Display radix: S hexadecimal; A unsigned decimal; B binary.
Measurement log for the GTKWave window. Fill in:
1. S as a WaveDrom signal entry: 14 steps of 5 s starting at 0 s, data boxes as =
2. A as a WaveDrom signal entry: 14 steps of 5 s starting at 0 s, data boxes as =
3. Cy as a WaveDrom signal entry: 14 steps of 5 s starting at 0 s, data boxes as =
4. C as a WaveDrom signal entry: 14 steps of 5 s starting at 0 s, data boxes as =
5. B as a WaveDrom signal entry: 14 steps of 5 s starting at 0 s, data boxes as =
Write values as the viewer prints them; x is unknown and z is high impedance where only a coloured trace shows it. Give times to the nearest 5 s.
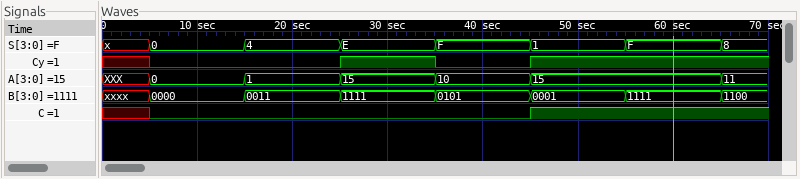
{name: 'S', wave: 'x=.=.=.=.=.=.=', data: '0 4 E F 1 F 8'}
{name: 'A', wave: 'x=.=.=.=.=...=', data: '0 1 15 10 15 11'}
{name: 'Cy', wave: 'x0...1.0.1....'}
{name: 'C', wave: 'x0.......1....'}
{name: 'B', wave: 'x=.=.=.=.=.=.=', data: '0000 0011 1111 0101 0001 1111 1100'}
